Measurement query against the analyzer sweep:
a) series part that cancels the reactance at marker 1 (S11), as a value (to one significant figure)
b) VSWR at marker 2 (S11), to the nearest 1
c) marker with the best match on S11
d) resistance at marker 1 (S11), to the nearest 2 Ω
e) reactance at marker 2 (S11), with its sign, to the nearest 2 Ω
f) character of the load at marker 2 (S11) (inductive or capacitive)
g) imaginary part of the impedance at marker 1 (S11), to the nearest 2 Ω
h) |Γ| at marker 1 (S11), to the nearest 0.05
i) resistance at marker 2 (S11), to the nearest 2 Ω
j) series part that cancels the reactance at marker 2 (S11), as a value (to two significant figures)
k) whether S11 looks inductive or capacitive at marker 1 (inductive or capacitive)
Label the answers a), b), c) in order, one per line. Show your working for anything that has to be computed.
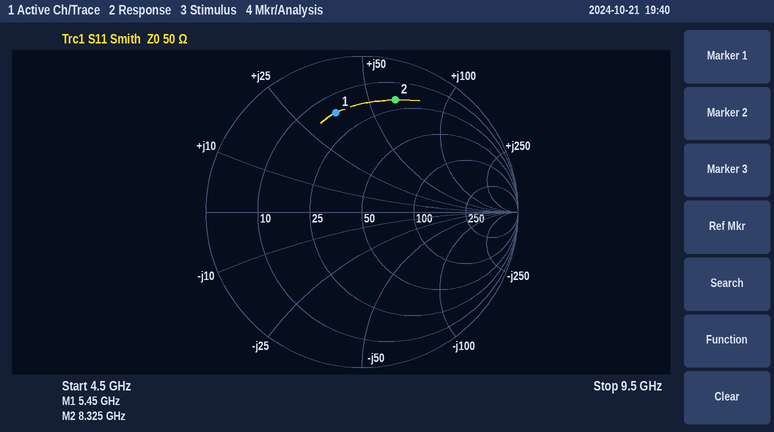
a) C = 1/(2π × 5.45 GHz × 36 Ω) ≈ 811 fF, so 800 fF to one significant figure
b) 7
c) marker 1
d) 16 Ω
e) +64 Ω
f) inductive
g) +36 Ω
h) 0.65
i) 20 Ω
j) C = 1/(2π × 8.325 GHz × 64 Ω) ≈ 299 fF, so 300 fF to two significant figures
k) inductive
